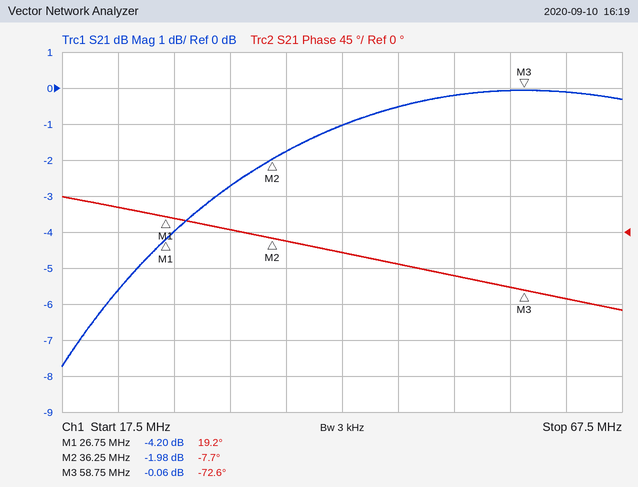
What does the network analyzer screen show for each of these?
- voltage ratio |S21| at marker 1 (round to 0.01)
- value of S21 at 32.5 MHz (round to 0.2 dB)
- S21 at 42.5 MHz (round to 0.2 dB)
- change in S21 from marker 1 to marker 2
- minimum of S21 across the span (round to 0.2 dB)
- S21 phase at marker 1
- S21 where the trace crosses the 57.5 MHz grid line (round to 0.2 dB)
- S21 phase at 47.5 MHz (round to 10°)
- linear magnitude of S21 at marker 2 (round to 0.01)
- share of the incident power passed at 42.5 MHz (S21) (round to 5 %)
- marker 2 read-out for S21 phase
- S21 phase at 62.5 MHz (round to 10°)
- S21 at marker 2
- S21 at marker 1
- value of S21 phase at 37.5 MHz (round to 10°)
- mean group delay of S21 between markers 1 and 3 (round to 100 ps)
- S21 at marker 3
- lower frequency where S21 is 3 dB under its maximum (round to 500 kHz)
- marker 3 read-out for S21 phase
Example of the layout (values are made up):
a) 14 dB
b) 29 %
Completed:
a) 0.62
b) -2.8 dB
c) -1.0 dB
d) 2.22 dB
e) -7.8 dB
f) 19.2°
g) 0.0 dB
h) -40°
i) 0.80
j) 80 %
k) -7.7°
l) -80°
m) -1.98 dB
n) -4.20 dB
o) -10°
p) 8.0 ns
q) -0.06 dB
r) 31.0 MHz
s) -72.6°
